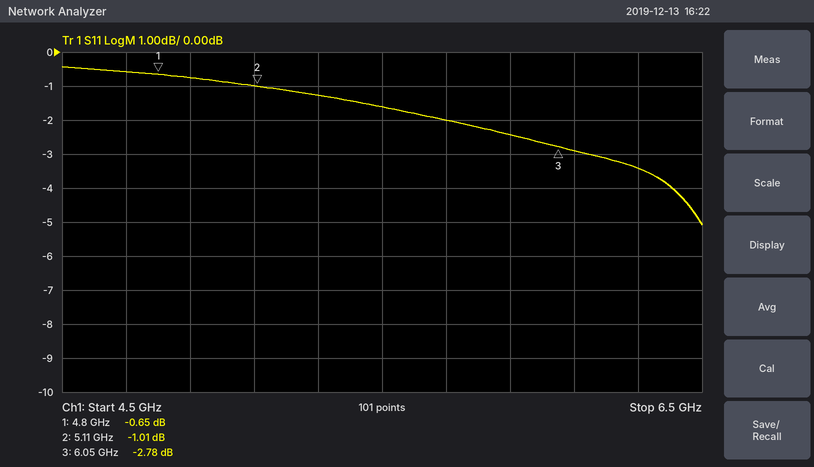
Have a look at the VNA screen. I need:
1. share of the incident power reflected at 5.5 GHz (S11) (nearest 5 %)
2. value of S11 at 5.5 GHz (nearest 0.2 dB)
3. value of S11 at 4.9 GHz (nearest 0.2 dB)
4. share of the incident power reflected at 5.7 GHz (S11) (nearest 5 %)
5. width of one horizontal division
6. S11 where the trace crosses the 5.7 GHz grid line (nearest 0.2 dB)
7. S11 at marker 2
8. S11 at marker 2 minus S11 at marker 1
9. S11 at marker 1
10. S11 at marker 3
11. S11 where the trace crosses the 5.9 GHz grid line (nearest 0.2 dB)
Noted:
70 %
-1.6 dB
-0.8 dB
65 %
200 MHz
-2.0 dB
-1.01 dB
-0.36 dB
-0.65 dB
-2.78 dB
-2.4 dB
